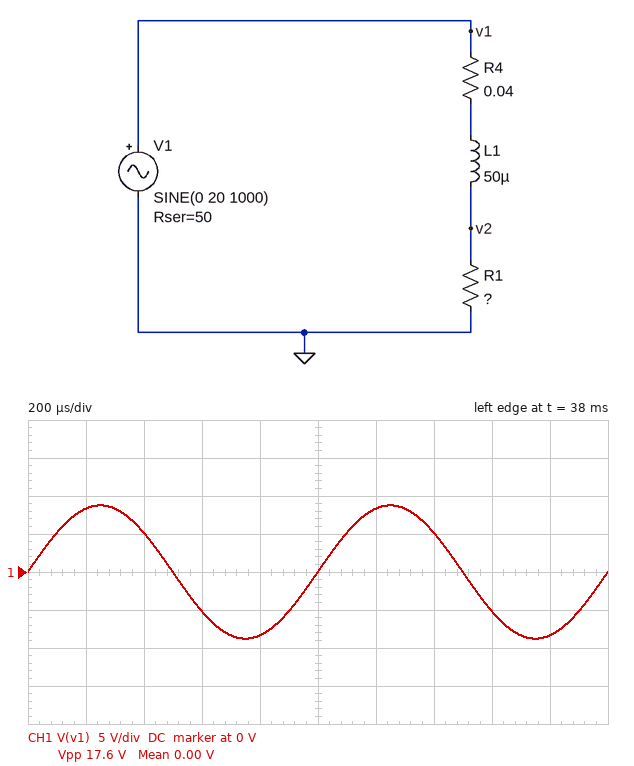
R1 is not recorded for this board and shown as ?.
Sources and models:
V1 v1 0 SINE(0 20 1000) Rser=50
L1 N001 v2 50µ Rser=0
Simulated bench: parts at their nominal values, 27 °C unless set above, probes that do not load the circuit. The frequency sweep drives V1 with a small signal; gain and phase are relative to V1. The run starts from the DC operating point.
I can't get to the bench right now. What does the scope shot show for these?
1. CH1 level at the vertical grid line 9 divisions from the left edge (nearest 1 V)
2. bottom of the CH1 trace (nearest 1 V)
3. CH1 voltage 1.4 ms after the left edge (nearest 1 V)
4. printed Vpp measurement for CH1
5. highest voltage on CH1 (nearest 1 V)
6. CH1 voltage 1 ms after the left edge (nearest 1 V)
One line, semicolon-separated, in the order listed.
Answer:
-8 V; -9 V; 5 V; 17.6 V; 9 V; 0 V
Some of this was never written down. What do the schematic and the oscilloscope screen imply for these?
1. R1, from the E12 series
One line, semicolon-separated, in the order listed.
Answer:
39 Ω
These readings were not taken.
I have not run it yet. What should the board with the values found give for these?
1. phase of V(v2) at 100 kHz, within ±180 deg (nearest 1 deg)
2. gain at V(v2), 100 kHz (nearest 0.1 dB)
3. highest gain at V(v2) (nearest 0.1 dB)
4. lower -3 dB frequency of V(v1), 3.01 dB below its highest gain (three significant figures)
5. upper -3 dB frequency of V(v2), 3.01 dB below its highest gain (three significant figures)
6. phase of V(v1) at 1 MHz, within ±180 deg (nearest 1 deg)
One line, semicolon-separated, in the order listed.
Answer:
-19 deg; -7.7 dB; -7.2 dB; 222 kHz; 283 kHz; 9 deg
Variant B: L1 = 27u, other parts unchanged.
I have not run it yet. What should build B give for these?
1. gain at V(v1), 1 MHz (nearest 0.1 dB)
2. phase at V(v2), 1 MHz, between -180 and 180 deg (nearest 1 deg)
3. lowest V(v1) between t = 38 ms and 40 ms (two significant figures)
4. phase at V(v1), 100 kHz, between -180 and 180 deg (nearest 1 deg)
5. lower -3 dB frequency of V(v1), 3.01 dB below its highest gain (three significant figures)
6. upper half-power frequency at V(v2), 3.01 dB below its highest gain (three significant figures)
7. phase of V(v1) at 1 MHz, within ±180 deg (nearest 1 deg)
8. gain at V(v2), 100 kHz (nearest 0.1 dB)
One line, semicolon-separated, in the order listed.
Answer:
-0.8 dB; -62 deg; -8.8 V; 13 deg; 412 kHz; 525 kHz; 15 deg; -7.3 dB
